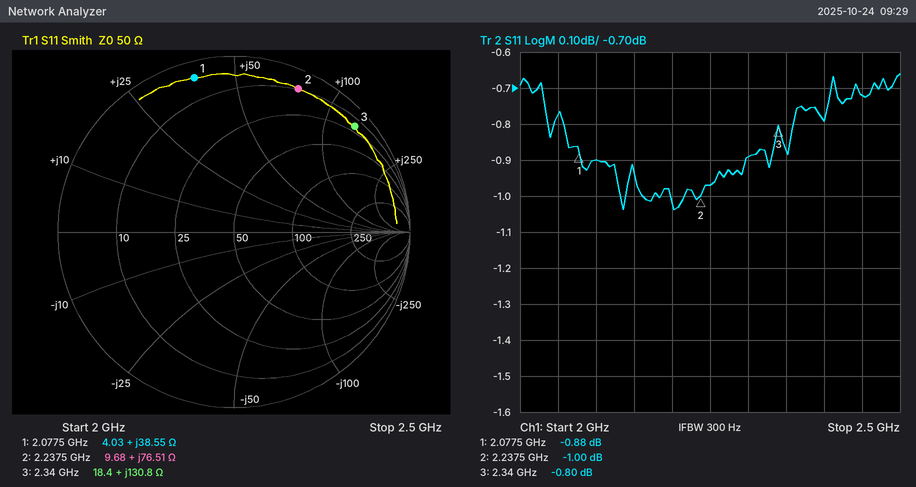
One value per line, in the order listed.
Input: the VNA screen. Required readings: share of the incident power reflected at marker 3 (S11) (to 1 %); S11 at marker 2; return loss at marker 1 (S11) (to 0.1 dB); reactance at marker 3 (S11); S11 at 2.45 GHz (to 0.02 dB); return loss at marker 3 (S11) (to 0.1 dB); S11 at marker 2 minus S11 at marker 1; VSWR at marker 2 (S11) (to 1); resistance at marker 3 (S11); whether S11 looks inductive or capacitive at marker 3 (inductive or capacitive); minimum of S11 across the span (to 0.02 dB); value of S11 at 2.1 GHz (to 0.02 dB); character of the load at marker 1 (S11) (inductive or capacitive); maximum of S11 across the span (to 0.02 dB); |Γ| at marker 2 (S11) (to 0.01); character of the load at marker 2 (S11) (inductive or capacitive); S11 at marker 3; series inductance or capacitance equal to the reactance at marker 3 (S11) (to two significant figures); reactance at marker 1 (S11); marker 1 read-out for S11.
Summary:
83 %
-1.00 dB
0.9 dB
+130.8 Ω
-0.72 dB
0.8 dB
-0.12 dB
17
18.4 Ω
inductive
-1.04 dB
-0.90 dB
inductive
-0.66 dB
0.89
inductive
-0.80 dB
8.9 nH
+38.55 Ω
-0.88 dB
